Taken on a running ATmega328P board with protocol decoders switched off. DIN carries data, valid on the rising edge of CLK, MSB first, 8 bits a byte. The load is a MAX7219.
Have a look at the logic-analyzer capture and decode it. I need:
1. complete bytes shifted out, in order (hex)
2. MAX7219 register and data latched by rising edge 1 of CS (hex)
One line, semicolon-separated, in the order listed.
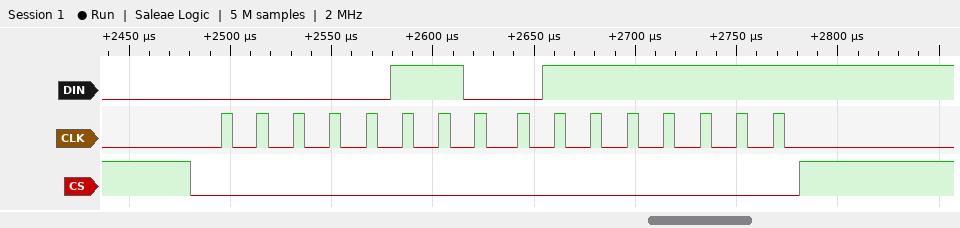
06 7F; register 0x6, data 0x7F
